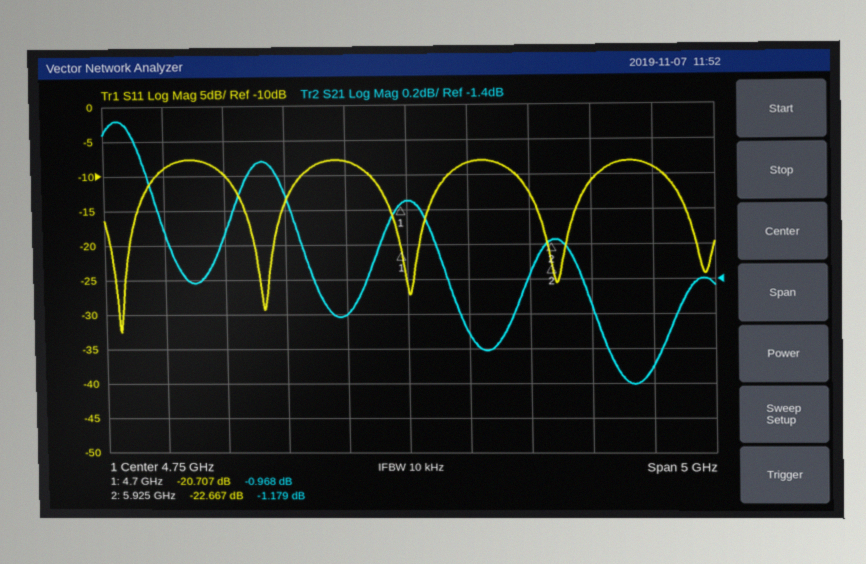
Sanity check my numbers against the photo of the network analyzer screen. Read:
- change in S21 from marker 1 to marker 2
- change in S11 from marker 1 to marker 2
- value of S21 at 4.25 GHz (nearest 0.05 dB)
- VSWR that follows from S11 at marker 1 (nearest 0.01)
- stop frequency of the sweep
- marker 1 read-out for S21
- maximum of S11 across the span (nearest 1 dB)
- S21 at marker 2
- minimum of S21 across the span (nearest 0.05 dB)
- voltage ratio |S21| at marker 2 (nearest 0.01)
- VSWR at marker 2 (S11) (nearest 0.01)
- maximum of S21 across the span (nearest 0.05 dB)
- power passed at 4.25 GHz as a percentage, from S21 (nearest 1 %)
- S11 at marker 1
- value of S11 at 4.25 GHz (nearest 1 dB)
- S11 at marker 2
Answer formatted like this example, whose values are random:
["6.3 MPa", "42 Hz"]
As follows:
["-0.211 dB", "-1.960 dB", "-1.60 dB", "1.20", "7.25 GHz", "-0.968 dB", "-8 dB", "-1.179 dB", "-2.00 dB", "0.87", "1.16", "-0.50 dB", "69 %", "-20.707 dB", "-8 dB", "-22.667 dB"]
